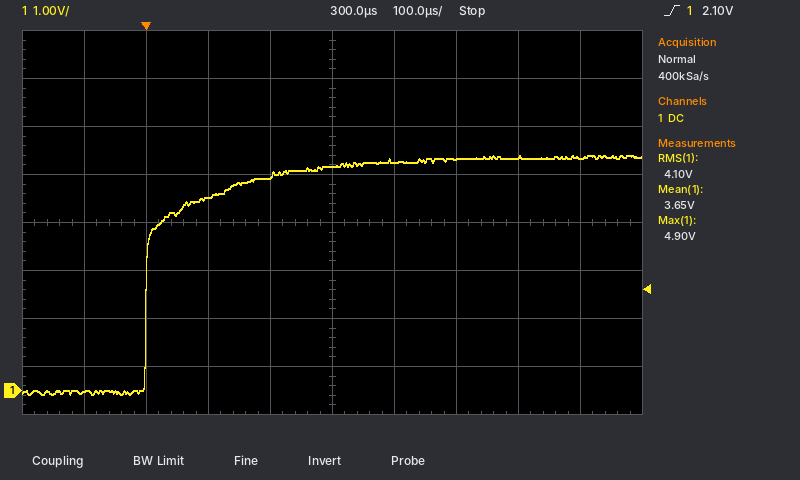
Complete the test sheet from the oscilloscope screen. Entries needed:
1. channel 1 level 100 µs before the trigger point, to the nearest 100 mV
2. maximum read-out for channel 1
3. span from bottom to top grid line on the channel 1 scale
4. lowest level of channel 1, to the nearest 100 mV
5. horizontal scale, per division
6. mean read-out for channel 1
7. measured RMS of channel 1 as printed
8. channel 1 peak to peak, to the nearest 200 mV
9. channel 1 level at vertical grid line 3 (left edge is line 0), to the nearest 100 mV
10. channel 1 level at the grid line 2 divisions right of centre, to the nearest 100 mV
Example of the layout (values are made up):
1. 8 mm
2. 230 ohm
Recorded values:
1. 0.0 V
2. 4.90 V
3. 8 V
4. -100 mV
5. 100 µs
6. 3.65 V
7. 4.10 V
8. 5.0 V
9. 4.0 V
10. 4.8 V
